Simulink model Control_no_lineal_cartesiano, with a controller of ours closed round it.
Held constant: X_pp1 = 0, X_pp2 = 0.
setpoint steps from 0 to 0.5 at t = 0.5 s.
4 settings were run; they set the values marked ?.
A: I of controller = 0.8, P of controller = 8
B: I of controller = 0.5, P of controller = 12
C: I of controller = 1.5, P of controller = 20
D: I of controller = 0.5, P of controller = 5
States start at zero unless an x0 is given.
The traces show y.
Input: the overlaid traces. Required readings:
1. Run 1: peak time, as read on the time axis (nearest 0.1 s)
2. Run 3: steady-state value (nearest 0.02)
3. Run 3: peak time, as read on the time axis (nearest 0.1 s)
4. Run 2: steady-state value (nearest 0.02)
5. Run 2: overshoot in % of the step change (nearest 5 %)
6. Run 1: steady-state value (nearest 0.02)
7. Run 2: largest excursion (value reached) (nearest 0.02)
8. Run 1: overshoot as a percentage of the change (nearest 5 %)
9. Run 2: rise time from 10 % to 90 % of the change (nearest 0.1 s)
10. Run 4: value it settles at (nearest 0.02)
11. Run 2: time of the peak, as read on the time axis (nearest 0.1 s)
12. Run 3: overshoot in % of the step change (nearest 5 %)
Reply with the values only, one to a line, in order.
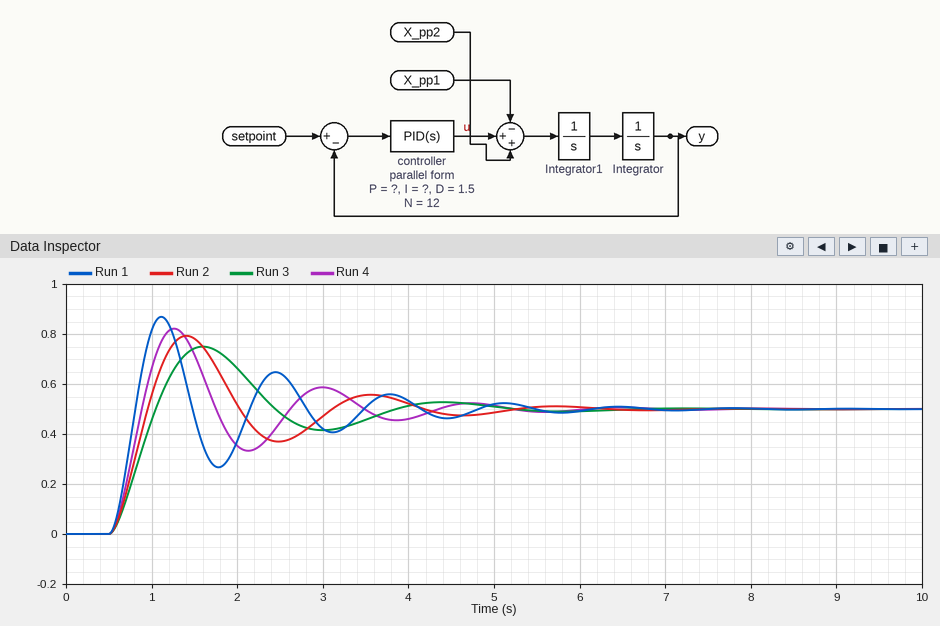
1.1 s
0.50
1.6 s
0.50
60 %
0.50
0.80
75 %
0.3 s
0.50
1.4 s
50 %
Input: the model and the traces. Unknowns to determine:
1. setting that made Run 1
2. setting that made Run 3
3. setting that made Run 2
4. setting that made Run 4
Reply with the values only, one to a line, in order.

C
D
A
B
